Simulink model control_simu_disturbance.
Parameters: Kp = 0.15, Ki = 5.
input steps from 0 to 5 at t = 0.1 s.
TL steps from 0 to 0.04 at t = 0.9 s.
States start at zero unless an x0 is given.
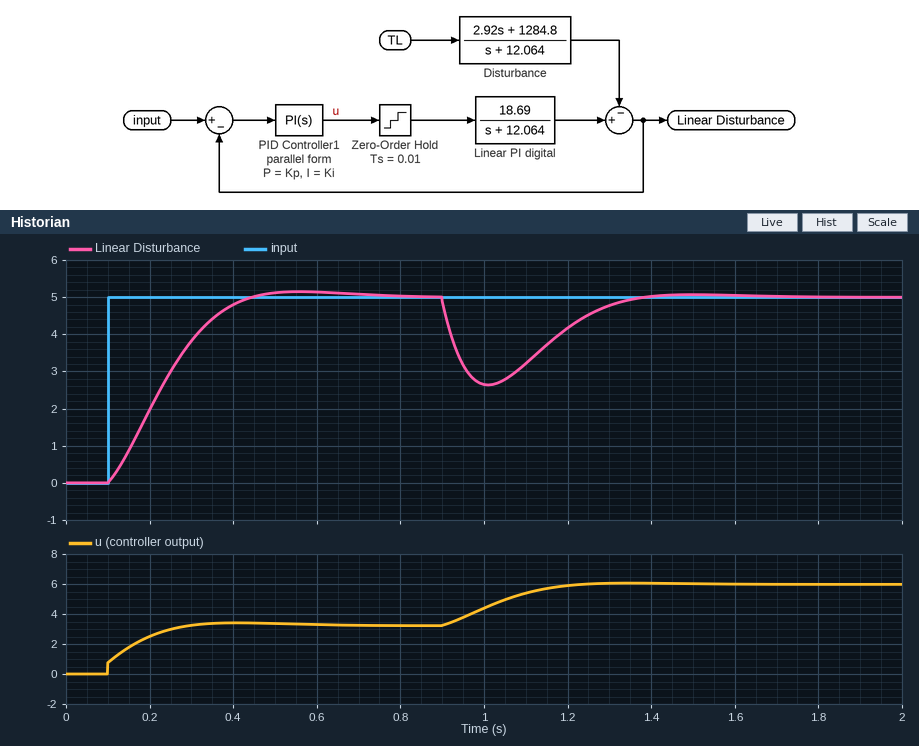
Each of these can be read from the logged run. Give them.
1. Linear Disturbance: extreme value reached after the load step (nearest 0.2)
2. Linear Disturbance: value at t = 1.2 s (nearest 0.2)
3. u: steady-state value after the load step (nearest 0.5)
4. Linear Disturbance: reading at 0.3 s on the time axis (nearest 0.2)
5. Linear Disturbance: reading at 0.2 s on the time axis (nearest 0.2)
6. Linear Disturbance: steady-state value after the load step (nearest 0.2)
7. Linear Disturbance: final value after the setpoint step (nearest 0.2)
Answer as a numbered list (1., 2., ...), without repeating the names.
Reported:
1. 2.6
2. 4.2
3. 6.0
4. 3.8
5. 2.0
6. 5.0
7. 5.0
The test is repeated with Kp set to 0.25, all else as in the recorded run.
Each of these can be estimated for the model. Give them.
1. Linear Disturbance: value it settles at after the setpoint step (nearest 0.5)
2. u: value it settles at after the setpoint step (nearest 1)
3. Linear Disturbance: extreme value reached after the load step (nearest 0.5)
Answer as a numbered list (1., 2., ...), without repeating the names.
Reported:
1. 5.0
2. 3
3. 3.0
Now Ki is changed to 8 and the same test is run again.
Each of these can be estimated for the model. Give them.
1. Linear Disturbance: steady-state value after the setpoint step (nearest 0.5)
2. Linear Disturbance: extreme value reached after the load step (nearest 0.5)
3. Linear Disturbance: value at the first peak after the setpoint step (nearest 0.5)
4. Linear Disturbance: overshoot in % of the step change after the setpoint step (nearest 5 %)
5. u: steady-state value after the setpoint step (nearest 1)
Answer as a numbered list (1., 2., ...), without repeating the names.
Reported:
1. 5.0
2. 3.0
3. 5.5
4. 10 %
5. 3
